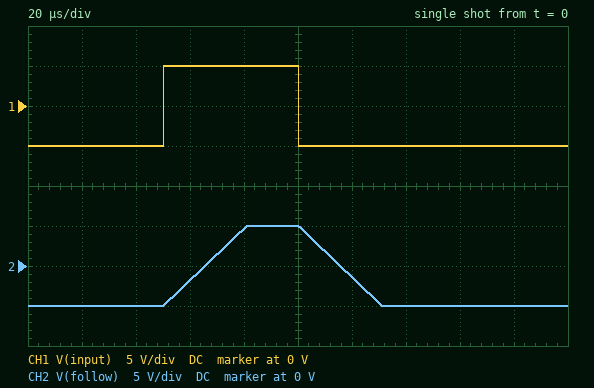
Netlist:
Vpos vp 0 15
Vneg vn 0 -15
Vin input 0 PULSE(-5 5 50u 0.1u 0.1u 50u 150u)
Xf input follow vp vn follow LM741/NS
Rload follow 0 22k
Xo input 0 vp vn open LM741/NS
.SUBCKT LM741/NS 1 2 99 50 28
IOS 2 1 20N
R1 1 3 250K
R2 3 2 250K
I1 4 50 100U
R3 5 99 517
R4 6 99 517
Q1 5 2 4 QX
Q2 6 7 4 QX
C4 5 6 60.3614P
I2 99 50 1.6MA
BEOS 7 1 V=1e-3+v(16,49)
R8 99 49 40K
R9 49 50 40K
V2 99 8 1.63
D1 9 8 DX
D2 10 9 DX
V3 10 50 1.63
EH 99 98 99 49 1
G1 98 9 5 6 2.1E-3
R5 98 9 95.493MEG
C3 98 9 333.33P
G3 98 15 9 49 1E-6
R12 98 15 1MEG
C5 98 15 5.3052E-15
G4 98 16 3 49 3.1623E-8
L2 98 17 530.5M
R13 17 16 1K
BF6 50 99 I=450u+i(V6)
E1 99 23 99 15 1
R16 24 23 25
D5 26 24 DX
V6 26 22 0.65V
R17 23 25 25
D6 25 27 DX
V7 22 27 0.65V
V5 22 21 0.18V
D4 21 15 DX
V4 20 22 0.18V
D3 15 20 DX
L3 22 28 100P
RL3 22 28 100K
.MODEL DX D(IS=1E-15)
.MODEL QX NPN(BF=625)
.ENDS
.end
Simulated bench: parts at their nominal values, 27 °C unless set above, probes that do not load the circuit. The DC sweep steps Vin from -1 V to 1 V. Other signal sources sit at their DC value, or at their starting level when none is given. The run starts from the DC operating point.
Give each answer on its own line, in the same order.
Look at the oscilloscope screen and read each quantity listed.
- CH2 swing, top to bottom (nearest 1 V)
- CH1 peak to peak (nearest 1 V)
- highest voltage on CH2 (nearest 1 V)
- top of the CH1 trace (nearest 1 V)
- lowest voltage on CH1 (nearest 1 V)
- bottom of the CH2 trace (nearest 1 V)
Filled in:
10 V
10 V
5 V
5 V
-5 V
-5 V
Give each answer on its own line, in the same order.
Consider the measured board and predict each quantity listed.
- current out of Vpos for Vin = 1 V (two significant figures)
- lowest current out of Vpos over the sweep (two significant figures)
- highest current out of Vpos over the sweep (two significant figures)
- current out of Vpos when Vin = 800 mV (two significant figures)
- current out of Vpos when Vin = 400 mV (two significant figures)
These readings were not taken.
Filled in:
3.4 mA
3.3 mA
3.4 mA
3.4 mA
3.4 mA
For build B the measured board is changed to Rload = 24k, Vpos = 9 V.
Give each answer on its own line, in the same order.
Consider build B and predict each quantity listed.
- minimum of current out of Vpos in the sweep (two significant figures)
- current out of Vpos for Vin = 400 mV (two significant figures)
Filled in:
3.1 mA
3.3 mA
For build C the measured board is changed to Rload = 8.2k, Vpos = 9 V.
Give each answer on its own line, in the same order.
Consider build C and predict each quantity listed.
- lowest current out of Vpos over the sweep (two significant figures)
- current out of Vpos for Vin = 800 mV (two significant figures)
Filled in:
3.1 mA
3.3 mA
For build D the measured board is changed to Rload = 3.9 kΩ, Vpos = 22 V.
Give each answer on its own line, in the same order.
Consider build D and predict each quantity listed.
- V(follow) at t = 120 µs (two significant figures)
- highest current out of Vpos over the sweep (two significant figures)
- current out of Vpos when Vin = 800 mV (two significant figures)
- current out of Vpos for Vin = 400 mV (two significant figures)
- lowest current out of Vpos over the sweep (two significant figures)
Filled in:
-1.3 V
3.8 mA
3.7 mA
3.6 mA
3.4 mA
